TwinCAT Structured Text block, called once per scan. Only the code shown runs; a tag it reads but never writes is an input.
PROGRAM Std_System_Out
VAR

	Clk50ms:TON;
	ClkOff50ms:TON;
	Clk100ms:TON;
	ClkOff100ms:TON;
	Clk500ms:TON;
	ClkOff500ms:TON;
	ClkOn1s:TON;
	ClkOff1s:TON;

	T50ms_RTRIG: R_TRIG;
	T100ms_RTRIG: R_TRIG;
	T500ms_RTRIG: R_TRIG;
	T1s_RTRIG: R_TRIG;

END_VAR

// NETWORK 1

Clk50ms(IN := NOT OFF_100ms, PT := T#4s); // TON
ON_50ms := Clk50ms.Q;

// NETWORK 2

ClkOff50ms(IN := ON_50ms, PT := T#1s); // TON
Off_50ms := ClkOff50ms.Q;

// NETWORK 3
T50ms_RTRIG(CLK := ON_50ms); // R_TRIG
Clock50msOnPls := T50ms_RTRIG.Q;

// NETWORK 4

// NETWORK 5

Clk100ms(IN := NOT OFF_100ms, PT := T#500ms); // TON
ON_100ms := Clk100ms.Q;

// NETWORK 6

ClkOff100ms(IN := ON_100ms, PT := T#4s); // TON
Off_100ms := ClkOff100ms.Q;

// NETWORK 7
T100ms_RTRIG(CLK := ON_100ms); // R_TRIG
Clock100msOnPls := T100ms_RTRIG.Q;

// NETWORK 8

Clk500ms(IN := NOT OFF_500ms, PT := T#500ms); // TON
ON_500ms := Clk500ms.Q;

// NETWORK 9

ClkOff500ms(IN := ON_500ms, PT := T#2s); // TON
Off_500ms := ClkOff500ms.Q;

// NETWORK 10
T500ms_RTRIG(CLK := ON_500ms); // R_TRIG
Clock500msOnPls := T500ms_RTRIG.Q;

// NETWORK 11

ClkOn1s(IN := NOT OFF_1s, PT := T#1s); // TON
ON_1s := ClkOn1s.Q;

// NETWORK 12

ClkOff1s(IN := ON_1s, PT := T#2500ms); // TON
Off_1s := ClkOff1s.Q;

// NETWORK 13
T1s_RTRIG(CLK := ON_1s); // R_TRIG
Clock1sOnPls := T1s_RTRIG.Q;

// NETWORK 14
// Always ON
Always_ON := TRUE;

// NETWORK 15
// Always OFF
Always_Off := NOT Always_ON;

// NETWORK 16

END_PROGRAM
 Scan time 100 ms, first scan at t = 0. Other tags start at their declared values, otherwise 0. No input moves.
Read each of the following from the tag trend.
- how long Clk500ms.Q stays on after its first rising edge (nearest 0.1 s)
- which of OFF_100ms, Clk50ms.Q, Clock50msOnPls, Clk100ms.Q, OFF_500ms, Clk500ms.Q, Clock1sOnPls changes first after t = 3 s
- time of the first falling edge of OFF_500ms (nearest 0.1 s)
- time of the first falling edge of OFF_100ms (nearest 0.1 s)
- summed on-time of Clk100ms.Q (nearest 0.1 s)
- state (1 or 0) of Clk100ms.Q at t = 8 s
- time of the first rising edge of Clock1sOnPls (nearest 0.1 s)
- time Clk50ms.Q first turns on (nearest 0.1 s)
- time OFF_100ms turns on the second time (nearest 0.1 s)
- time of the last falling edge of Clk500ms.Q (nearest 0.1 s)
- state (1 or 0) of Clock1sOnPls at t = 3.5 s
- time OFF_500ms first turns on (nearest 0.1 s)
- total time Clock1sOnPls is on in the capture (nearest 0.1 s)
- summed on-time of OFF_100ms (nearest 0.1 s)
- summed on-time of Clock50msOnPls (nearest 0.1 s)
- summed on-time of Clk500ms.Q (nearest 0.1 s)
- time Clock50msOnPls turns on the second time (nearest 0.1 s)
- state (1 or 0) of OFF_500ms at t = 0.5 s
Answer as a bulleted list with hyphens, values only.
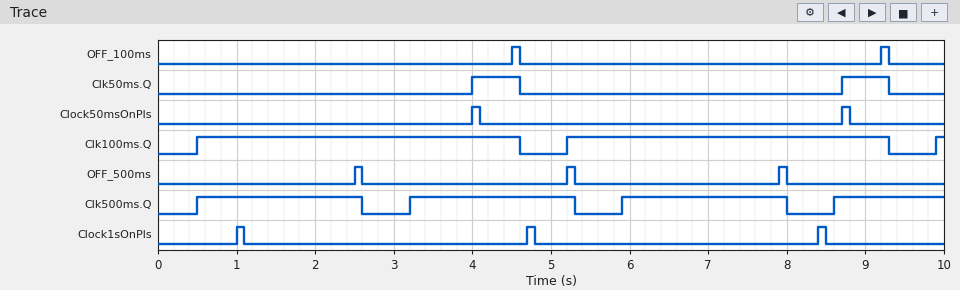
- 2.1 s
- Clk500ms.Q
- 2.6 s
- 4.6 s
- 8.3 s
- 1
- 1.0 s
- 4.0 s
- 9.2 s
- 8.0 s
- 0
- 2.5 s
- 0.3 s
- 0.2 s
- 0.2 s
- 7.7 s
- 8.7 s
- 0
